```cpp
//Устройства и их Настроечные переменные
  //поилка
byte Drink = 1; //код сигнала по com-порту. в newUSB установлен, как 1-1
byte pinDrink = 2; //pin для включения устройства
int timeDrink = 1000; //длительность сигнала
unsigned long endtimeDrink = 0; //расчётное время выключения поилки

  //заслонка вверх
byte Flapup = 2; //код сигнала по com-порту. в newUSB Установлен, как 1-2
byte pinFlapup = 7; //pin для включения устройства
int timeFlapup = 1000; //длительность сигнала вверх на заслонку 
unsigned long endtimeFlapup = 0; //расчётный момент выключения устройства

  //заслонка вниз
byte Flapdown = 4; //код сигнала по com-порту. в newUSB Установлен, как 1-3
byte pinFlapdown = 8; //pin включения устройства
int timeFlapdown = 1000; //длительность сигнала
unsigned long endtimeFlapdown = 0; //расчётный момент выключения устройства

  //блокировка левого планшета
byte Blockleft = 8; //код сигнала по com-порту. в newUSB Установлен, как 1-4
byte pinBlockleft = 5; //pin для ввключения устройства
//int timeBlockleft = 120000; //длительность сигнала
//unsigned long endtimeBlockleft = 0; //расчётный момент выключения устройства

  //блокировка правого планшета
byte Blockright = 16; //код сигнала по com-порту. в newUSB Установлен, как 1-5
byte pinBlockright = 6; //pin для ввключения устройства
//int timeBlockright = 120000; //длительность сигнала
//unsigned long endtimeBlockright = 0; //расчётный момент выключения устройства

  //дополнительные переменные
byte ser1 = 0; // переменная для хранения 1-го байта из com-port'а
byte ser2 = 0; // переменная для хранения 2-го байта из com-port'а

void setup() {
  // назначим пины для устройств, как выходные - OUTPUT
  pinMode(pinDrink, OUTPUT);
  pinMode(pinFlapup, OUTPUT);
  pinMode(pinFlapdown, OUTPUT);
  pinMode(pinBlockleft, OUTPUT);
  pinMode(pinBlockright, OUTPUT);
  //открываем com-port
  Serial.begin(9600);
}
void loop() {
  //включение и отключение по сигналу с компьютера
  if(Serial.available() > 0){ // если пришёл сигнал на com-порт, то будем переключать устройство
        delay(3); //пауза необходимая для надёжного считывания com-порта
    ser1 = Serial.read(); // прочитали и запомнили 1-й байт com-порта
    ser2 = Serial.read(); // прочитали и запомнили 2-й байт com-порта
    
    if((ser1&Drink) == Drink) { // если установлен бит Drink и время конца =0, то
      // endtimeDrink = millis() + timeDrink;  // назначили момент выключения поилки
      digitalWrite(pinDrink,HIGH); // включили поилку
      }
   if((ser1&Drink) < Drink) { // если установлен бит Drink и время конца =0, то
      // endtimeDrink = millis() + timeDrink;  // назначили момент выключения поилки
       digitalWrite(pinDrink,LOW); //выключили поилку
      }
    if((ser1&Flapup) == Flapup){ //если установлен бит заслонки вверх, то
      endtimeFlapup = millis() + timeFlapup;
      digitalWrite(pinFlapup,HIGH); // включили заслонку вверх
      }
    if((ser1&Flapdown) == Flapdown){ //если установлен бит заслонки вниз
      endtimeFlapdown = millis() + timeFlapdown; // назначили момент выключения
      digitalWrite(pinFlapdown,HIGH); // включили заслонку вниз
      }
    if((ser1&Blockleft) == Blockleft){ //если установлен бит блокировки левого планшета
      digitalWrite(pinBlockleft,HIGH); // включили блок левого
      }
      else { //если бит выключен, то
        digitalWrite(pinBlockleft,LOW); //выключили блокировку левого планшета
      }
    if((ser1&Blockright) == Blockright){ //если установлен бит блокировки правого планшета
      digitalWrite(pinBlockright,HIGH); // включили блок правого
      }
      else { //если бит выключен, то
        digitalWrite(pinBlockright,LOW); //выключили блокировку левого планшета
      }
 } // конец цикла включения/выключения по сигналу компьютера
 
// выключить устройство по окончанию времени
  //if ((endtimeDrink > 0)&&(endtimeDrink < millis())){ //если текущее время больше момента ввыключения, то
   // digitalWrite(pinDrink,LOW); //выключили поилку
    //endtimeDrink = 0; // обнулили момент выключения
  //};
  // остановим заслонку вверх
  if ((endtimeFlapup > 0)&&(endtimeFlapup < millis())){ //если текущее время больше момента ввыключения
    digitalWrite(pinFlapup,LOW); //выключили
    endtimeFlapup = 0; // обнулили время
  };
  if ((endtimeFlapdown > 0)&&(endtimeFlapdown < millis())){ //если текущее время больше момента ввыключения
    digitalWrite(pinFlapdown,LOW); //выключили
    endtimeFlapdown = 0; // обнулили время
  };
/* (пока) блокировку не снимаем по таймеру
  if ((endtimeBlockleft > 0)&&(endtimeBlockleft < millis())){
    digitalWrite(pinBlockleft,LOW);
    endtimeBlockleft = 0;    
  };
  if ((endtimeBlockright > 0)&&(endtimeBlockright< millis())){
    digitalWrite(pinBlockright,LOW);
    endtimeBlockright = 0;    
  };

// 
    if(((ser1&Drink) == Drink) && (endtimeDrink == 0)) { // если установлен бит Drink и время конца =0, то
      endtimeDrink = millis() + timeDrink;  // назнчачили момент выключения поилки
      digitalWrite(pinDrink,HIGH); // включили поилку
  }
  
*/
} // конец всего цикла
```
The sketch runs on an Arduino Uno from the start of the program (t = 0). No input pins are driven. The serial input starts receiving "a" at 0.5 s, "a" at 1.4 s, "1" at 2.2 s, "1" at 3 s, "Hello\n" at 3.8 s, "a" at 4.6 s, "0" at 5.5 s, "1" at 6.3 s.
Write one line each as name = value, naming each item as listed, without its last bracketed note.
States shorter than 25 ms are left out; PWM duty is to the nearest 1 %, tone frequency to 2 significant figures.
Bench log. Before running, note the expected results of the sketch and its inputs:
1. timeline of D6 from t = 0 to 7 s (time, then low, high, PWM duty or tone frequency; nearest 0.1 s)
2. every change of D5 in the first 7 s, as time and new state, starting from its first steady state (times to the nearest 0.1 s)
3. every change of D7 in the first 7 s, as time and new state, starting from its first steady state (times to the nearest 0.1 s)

timeline of D6 from t = 0 to 7 s = 0 s low; 2.2 s high; 3.8 s low; 5.5 s high
every change of D5 in the first 7 s, as time and new state, starting from its first steady state = 0 s low; 3.8 s high; 4.6 s low
every change of D7 in the first 7 s, as time and new state, starting from its first steady state = 0 s low; 3.8 s high; 4.8 s low
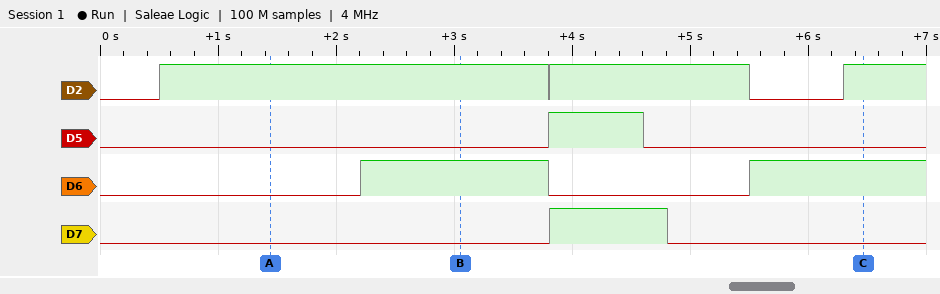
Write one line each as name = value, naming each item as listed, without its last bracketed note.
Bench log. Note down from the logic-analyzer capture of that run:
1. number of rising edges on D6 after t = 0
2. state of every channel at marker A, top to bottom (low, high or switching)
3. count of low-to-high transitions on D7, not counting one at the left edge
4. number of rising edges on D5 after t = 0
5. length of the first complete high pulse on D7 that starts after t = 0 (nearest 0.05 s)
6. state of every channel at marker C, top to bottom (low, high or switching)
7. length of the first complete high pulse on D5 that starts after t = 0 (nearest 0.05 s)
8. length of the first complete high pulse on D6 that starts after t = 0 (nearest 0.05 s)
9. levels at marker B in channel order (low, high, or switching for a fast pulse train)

number of rising edges on D6 after t = 0 = 2
state of every channel at marker A, top to bottom = D2 high, D5 low, D6 low, D7 low
count of low-to-high transitions on D7, not counting one at the left edge = 1
number of rising edges on D5 after t = 0 = 1
length of the first complete high pulse on D7 that starts after t = 0 = 1.00 s
state of every channel at marker C, top to bottom = D2 high, D5 low, D6 high, D7 low
length of the first complete high pulse on D5 that starts after t = 0 = 0.80 s
length of the first complete high pulse on D6 that starts after t = 0 = 1.60 s
levels at marker B in channel order = D2 high, D5 low, D6 high, D7 low
